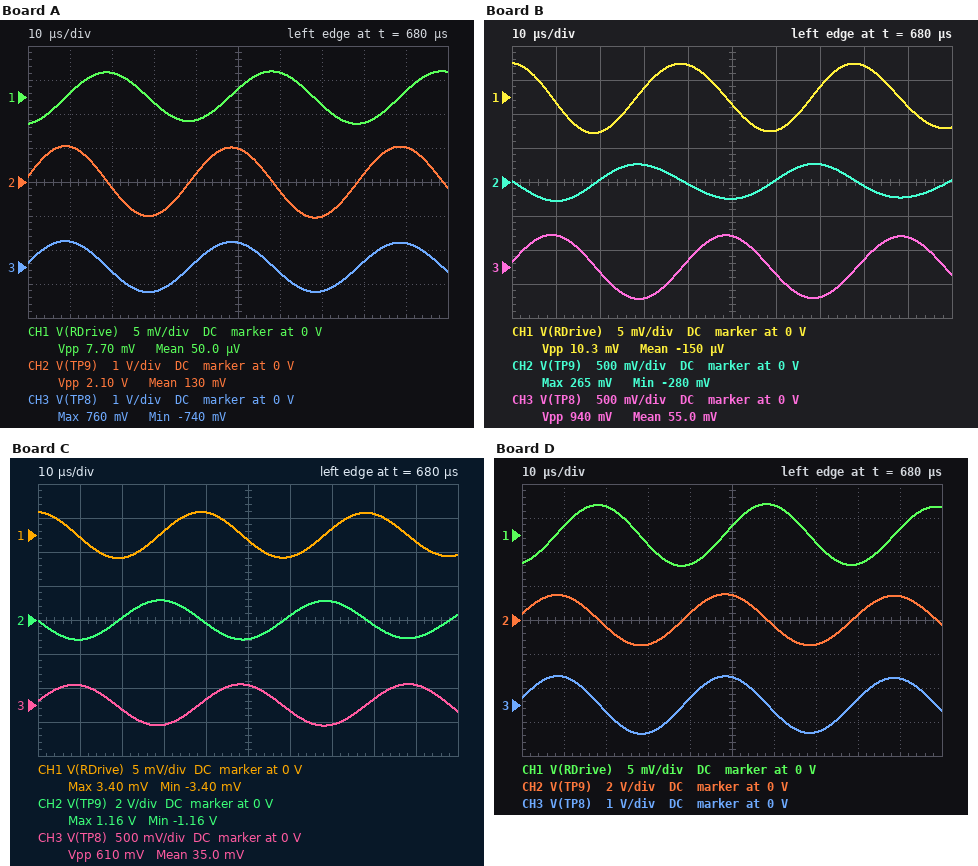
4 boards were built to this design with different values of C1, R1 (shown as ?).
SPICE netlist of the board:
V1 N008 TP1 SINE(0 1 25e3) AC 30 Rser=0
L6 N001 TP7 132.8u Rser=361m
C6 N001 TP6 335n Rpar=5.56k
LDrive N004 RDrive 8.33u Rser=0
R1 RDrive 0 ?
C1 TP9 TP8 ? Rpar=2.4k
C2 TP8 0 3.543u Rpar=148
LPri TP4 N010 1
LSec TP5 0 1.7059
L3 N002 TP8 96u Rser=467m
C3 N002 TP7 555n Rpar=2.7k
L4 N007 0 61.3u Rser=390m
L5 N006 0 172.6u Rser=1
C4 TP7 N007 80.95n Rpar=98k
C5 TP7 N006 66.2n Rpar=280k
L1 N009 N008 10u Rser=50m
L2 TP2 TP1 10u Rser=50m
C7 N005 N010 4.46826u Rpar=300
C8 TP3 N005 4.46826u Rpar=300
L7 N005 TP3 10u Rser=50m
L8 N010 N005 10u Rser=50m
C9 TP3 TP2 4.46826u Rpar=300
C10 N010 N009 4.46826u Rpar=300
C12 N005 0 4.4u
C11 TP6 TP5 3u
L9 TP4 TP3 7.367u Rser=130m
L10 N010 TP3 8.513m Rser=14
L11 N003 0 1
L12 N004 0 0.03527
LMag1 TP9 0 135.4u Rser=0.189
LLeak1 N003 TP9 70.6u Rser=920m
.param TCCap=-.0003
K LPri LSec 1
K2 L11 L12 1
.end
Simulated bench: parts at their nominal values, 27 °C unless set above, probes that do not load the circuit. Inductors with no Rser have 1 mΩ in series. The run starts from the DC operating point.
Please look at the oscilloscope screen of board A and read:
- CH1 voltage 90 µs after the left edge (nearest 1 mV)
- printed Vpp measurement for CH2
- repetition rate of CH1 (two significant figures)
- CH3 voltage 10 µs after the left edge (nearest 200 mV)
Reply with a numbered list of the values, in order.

1. 1 mV
2. 2.10 V
3. 25 kHz
4. 800 mV
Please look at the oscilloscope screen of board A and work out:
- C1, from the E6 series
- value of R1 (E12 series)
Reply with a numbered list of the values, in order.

1. 1.5 µF
2. 0.033 Ω
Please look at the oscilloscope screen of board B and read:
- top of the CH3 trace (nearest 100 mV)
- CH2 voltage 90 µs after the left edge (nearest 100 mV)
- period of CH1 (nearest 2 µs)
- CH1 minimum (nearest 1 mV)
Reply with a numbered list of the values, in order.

1. 500 mV
2. -200 mV
3. 40 µs
4. -5 mV
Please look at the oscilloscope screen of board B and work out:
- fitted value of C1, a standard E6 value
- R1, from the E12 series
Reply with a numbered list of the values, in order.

1. 150 nF
2. 0.18 Ω
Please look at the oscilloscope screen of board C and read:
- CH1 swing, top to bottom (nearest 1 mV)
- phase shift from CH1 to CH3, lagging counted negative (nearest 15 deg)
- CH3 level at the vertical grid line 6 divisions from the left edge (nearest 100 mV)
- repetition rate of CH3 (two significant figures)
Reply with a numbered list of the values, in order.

1. 7 mV
2. -90 deg
3. -100 mV
4. 25 kHz
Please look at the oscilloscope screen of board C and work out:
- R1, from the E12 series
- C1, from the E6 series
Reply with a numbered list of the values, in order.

1. 0.027 Ω
2. 330 nF
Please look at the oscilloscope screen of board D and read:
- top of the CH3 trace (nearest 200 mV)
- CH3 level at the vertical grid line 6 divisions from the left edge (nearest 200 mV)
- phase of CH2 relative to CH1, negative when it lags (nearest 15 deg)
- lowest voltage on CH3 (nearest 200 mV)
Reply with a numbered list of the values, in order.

1. 800 mV
2. -200 mV
3. 90 deg
4. -800 mV
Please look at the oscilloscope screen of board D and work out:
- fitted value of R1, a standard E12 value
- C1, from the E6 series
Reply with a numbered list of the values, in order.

1. 0.027 Ω
2. 1 µF
